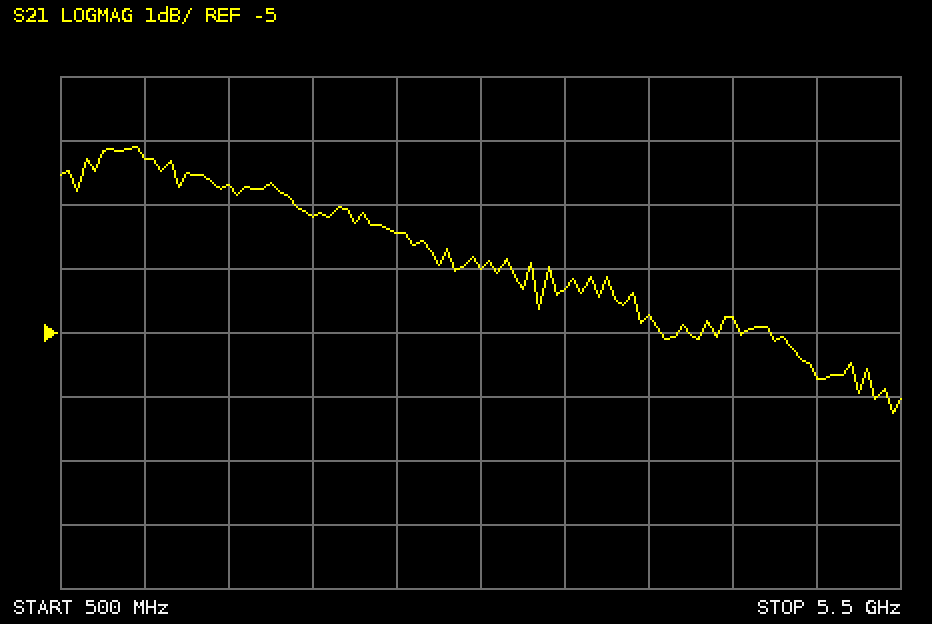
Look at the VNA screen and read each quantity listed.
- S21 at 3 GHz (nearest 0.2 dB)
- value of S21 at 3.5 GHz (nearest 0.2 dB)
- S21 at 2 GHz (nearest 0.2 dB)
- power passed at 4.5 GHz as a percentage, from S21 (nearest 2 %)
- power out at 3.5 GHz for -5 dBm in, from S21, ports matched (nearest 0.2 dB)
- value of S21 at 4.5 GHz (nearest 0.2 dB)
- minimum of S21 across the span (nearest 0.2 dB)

-4.0 dB
-4.4 dB
-3.2 dB
34 %
-9.4 dBm
-4.8 dB
-6.2 dB
